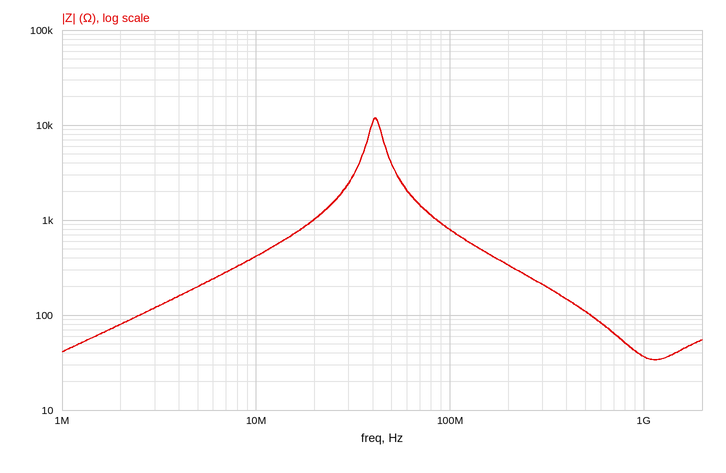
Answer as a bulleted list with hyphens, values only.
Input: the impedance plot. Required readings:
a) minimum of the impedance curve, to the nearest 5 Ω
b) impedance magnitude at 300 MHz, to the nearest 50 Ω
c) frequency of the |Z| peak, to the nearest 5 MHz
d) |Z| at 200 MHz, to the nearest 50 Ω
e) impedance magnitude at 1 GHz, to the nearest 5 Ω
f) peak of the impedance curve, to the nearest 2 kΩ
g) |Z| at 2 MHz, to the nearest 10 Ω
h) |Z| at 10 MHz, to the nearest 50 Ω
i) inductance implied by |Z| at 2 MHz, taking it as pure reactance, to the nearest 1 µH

- 35 Ω
- 200 Ω
- 40 MHz
- 350 Ω
- 35 Ω
- 12 kΩ
- 80 Ω
- 400 Ω
- 6 µH
